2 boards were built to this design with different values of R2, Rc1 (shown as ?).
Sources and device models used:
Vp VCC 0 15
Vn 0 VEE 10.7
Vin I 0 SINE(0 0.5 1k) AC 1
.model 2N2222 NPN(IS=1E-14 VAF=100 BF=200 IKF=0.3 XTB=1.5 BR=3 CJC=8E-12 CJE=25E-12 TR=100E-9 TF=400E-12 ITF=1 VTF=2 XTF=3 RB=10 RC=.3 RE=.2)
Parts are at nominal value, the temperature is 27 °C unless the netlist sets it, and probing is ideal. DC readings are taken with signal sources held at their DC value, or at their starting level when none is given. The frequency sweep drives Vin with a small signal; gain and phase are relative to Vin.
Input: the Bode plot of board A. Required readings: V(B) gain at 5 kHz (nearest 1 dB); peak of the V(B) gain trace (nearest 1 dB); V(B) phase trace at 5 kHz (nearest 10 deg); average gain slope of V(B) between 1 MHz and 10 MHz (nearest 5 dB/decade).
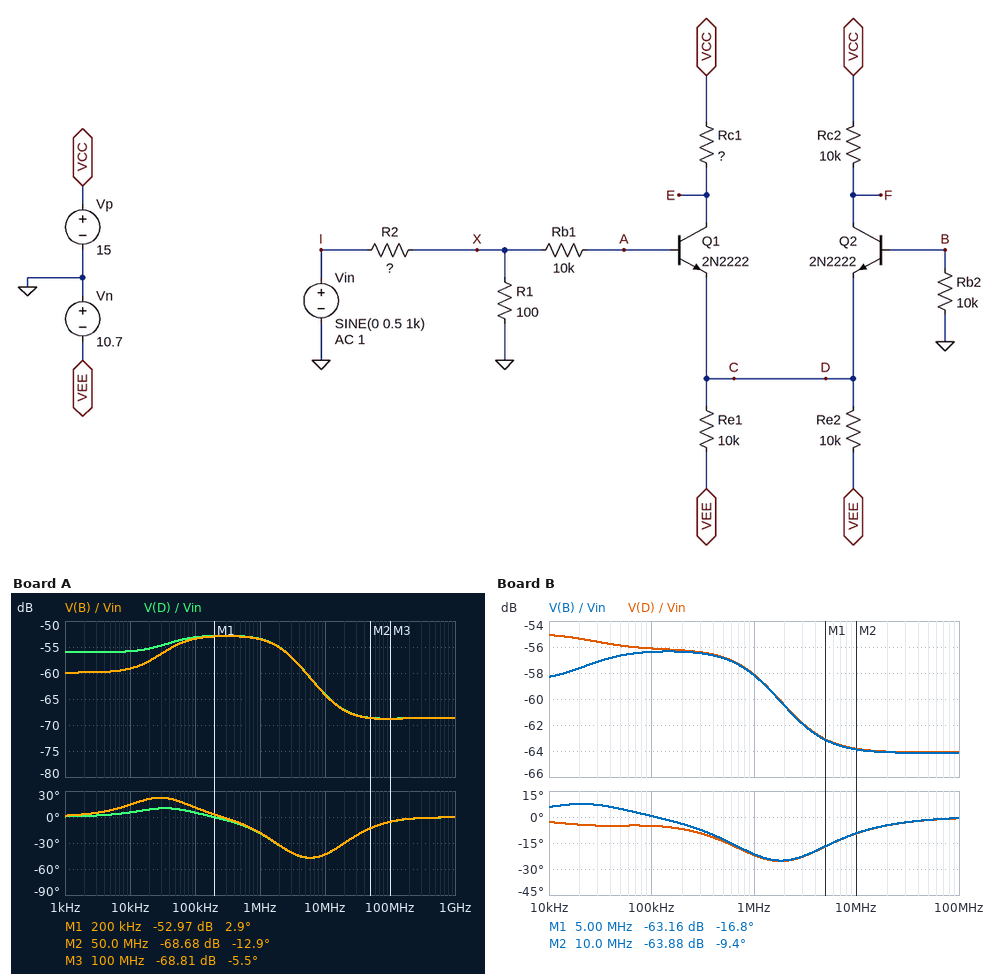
-60 dB
-53 dB
10 deg
-10 dB/decade
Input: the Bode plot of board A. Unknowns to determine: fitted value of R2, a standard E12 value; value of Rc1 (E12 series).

33 kΩ
3.3 kΩ
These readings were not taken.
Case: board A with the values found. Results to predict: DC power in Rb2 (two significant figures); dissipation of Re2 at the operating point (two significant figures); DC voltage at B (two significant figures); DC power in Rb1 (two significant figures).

210 nW
10 mW
-46 mV
210 nW
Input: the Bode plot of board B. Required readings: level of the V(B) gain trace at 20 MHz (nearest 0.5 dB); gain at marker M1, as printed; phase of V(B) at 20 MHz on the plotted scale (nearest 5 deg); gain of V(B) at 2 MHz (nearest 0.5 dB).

-64.0 dB
-63.16 dB
-5 deg
-60.5 dB
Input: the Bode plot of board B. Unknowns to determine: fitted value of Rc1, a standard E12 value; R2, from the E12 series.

12 kΩ
27 kΩ
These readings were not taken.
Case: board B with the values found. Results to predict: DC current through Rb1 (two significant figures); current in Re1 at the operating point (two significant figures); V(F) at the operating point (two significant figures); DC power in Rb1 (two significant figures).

4.8 µA
1.0 mA
4.9 V
230 nW
